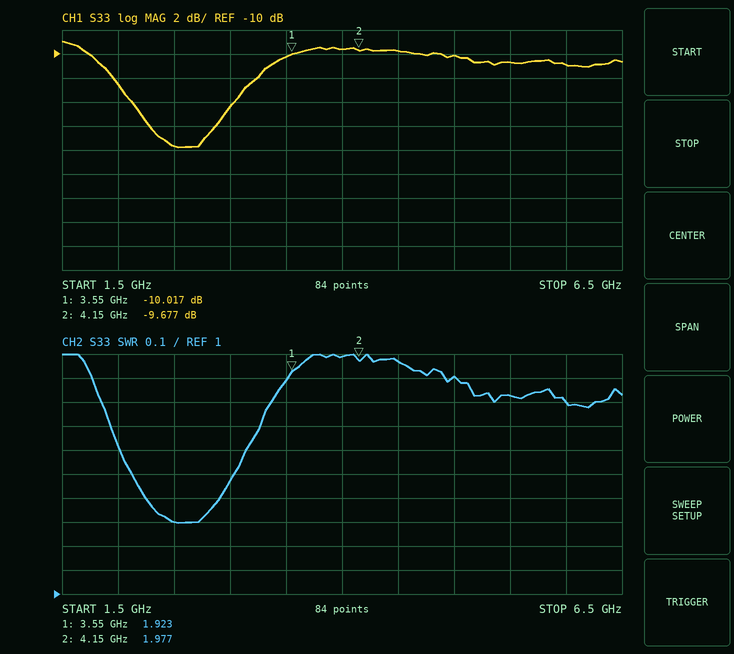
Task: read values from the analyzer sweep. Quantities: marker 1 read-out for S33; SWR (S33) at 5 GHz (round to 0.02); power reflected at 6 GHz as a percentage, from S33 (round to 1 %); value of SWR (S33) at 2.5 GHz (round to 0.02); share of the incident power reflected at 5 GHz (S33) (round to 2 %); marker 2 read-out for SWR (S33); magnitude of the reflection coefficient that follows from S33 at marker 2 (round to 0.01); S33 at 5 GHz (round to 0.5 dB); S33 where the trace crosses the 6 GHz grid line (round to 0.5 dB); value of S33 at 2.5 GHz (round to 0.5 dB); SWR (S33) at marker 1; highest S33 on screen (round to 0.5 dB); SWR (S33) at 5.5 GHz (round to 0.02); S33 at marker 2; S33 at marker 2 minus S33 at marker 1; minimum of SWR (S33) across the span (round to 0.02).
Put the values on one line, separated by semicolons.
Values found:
-10.017 dB; 1.90; 8 %; 1.30; 10 %; 1.977; 0.33; -10.0 dB; -11.0 dB; -17.5 dB; 1.923; -9.0 dB; 1.82; -9.677 dB; 0.340 dB; 1.30
